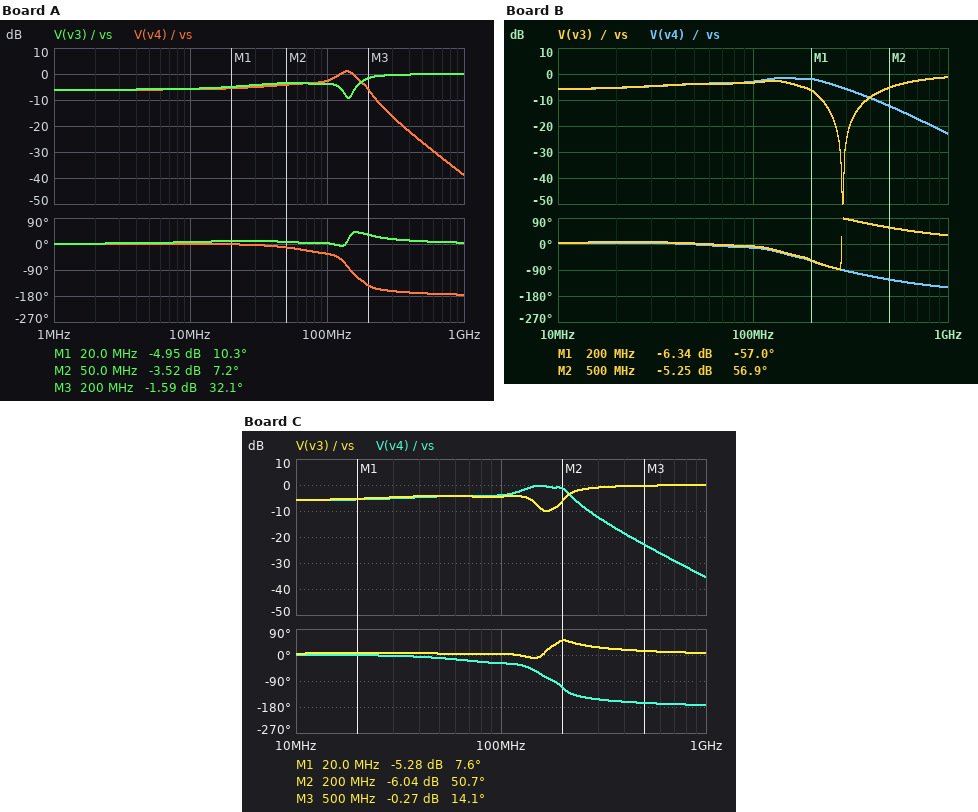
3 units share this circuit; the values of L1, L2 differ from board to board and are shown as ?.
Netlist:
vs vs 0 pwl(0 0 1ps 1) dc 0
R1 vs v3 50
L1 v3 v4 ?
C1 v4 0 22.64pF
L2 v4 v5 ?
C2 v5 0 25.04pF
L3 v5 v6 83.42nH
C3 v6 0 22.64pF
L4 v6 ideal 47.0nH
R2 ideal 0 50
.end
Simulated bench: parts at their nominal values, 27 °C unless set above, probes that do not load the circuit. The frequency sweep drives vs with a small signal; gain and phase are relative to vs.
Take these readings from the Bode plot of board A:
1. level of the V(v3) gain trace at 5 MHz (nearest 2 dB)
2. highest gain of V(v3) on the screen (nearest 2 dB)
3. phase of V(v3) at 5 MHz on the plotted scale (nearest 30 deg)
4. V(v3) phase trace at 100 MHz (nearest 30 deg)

-6 dB
0 dB
0 deg
0 deg
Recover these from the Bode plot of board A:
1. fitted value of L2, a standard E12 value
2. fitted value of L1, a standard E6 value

150 nH
100 nH
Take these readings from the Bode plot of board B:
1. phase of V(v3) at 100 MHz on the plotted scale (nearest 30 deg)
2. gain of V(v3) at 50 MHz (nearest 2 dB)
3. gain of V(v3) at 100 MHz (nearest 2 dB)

0 deg
-4 dB
-4 dB
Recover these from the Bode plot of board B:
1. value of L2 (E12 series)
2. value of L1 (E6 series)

150 nH
15 nH
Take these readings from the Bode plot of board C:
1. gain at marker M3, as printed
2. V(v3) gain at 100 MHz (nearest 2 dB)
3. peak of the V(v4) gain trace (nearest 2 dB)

-0.27 dB
-4 dB
0 dB
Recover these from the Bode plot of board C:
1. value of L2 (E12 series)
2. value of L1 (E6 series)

120 nH
68 nH
